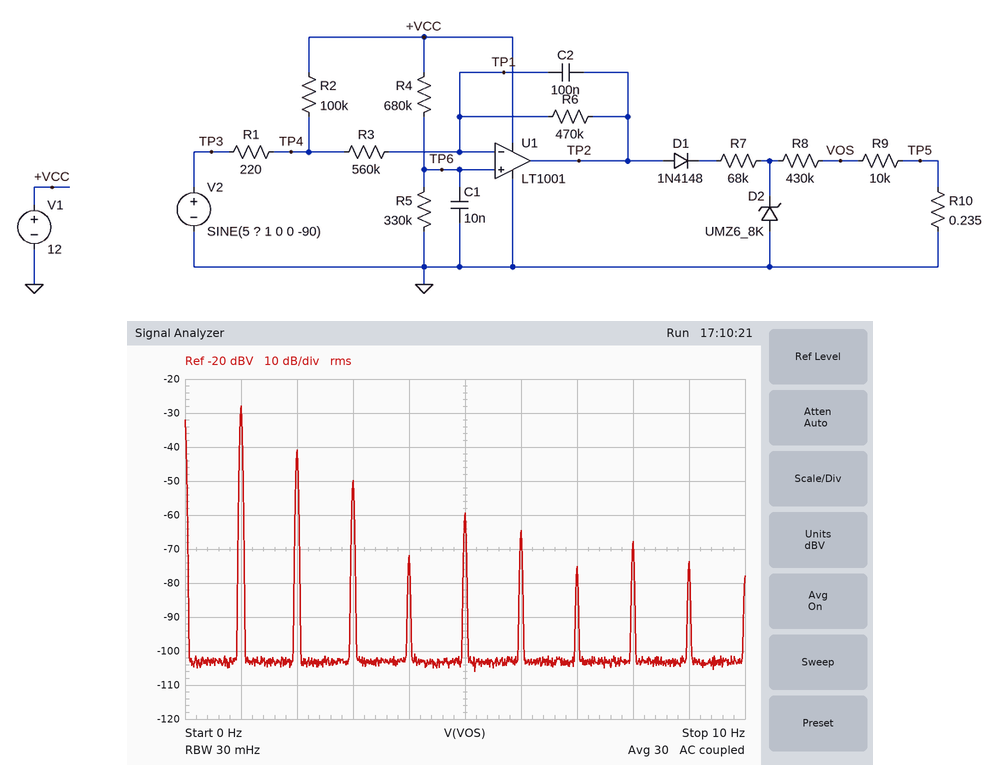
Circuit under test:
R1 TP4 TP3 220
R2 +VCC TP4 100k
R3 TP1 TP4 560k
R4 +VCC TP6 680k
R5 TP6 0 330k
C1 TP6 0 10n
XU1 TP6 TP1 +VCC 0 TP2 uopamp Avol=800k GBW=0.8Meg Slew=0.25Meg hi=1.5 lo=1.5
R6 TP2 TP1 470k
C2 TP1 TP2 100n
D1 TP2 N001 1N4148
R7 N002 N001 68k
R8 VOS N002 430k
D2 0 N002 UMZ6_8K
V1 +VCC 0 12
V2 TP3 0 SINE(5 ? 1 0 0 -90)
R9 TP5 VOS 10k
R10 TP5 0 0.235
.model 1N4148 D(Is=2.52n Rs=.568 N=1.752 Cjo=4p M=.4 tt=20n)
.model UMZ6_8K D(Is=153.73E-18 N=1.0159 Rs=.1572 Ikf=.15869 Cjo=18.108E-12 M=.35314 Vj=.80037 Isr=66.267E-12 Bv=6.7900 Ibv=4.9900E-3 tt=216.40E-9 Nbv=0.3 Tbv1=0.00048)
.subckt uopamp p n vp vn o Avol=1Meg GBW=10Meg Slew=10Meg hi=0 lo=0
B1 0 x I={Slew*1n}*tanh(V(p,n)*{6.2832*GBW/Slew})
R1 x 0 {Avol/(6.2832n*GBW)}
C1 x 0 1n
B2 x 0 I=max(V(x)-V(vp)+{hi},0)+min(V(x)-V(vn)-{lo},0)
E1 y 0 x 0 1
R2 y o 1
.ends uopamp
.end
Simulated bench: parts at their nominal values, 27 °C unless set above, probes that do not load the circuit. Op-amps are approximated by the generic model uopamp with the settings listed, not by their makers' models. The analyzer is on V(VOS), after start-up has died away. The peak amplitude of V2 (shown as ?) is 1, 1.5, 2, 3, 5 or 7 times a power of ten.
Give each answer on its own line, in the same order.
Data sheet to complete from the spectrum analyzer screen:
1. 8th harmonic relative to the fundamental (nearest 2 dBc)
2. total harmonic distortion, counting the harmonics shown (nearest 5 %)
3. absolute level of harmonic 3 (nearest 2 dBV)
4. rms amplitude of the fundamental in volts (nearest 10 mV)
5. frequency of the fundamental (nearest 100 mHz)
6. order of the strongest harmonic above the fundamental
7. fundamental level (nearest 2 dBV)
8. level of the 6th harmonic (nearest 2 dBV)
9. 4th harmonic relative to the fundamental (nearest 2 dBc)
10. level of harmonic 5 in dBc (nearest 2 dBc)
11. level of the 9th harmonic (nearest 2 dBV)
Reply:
-40 dBc
25 %
-50 dBV
40 mV
1.0 Hz
2
-28 dBV
-64 dBV
-44 dBc
-32 dBc
-74 dBV
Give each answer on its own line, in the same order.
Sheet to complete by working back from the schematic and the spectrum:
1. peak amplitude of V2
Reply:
5 V
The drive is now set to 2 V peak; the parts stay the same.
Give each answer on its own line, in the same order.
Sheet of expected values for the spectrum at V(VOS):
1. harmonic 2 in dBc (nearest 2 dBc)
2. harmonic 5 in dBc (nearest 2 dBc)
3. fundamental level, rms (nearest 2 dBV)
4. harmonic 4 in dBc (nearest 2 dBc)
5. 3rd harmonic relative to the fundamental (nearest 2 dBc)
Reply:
-38 dBc
-44 dBc
-34 dBV
-42 dBc
-40 dBc
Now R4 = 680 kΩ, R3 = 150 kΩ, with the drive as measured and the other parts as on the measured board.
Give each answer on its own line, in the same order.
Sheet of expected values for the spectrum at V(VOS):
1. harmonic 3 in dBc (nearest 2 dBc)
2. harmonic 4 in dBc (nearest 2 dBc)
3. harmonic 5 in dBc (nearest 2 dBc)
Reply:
-14 dBc
-14 dBc
-30 dBc
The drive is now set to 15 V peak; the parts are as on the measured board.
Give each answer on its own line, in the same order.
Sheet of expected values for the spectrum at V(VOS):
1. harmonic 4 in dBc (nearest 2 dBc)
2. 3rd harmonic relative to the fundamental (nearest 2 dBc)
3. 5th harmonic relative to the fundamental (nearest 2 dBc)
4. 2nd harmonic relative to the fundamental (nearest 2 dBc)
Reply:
-20 dBc
-12 dBc
-20 dBc
-18 dBc
